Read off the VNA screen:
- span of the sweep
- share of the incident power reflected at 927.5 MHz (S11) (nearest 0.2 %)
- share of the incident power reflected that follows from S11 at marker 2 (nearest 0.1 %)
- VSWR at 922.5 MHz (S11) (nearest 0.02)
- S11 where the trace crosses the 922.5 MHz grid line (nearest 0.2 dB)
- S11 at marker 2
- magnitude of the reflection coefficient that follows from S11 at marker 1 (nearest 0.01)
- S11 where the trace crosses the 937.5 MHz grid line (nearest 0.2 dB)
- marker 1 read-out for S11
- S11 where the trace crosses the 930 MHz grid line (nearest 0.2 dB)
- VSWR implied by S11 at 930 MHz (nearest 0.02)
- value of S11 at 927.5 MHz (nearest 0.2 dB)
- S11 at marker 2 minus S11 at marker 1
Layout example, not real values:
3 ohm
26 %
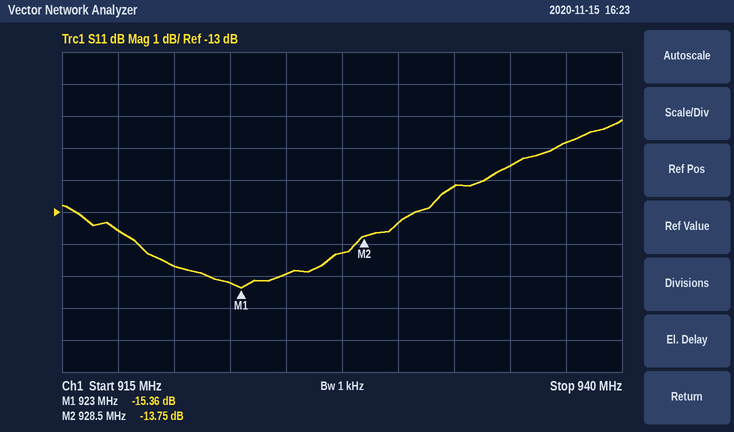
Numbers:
25 MHz
3.8 %
4.2 %
1.42
-15.2 dB
-13.75 dB
0.17
-10.8 dB
-15.36 dB
-13.4 dB
1.54
-14.2 dB
1.61 dB
